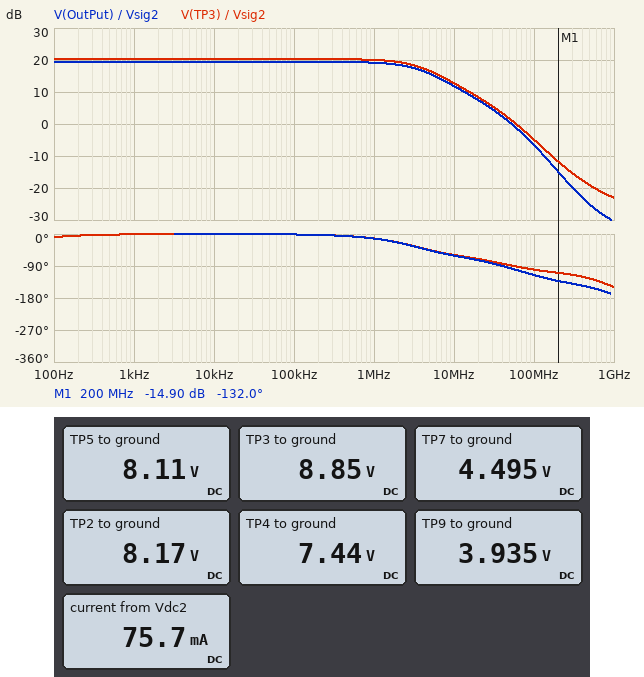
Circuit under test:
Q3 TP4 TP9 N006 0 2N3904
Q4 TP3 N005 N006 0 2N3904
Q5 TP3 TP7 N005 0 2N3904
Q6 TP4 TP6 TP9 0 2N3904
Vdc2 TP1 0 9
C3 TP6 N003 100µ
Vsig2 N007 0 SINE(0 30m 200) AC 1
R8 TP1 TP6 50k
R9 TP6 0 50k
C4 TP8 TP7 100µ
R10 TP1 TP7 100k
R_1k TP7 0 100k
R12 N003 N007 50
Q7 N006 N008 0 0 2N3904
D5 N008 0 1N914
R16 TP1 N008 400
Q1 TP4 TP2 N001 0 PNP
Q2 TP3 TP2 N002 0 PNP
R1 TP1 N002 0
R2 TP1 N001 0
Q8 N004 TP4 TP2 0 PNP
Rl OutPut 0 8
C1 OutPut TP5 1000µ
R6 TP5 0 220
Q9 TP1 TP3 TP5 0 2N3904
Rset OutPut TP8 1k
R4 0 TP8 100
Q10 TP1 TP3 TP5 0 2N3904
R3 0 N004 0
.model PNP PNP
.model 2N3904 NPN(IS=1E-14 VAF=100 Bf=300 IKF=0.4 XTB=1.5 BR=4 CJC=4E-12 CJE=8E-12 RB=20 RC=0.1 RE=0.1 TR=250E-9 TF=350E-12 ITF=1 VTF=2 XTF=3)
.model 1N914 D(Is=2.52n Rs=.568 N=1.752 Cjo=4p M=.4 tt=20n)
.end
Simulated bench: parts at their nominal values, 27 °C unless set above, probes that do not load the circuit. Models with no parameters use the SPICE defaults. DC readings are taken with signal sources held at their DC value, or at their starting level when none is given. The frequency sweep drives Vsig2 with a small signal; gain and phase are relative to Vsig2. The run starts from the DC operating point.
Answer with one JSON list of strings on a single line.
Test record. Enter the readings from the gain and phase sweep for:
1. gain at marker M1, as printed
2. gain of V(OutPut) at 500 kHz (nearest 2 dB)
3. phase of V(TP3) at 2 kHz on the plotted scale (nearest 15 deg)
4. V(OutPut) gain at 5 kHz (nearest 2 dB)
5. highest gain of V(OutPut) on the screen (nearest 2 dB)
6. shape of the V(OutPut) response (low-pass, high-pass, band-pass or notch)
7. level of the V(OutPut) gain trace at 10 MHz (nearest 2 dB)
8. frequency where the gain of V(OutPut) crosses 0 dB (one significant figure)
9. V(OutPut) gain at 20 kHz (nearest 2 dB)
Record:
["-14.90 dB", "20 dB", "0 deg", "20 dB", "20 dB", "low-pass", "12 dB", "50 MHz", "20 dB"]
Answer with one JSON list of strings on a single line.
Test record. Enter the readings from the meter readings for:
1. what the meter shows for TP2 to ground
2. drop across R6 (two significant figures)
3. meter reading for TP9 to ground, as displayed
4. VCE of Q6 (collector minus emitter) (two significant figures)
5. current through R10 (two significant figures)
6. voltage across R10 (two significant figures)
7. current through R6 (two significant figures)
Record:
["8.17 V", "8.1 V", "3.935 V", "3.5 V", "45 µA", "4.5 V", "37 mA"]
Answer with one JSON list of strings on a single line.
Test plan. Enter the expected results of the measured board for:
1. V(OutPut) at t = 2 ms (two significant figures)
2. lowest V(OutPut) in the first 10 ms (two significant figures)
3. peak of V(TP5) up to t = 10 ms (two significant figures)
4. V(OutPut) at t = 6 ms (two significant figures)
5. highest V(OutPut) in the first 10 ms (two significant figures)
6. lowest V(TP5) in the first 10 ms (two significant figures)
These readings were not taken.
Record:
["67 mV", "-280 mV", "8.2 V", "120 mV", "120 mV", "7.8 V"]
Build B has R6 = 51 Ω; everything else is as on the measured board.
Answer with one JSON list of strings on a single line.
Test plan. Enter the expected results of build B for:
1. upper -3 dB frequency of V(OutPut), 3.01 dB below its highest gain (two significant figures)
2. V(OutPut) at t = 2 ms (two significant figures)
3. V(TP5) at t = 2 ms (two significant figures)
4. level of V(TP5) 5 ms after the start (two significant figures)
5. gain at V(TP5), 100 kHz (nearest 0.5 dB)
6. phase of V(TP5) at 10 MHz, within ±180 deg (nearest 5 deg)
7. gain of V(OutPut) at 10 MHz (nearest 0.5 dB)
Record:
["4.8 MHz", "180 mV", "6.3 V", "6.0 V", "20.5 dB", "-65 deg", "13.5 dB"]
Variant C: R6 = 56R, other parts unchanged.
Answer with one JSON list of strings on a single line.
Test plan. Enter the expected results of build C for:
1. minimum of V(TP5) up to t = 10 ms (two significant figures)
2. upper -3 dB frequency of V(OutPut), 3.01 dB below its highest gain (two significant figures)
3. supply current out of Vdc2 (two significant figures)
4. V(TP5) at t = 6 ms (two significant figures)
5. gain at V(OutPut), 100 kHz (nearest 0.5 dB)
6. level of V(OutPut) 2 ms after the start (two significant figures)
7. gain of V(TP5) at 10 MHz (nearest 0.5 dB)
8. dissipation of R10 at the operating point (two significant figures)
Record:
["6.0 V", "4.9 MHz", "150 mA", "6.6 V", "20.5 dB", "180 mV", "13.5 dB", "200 µW"]
